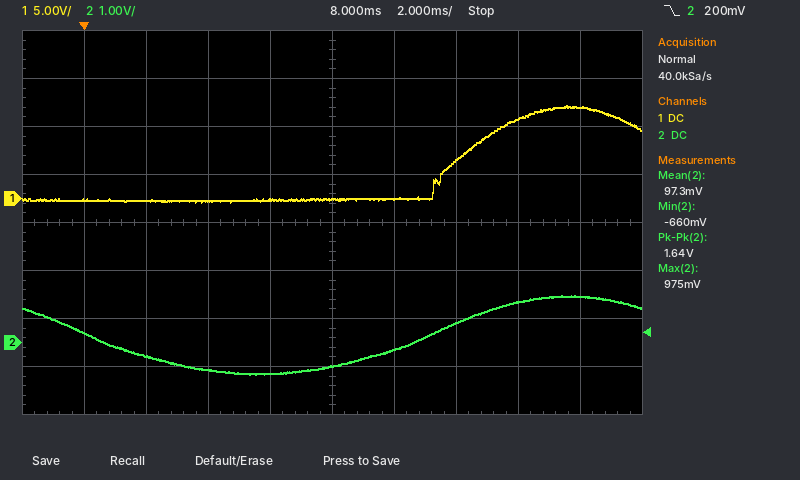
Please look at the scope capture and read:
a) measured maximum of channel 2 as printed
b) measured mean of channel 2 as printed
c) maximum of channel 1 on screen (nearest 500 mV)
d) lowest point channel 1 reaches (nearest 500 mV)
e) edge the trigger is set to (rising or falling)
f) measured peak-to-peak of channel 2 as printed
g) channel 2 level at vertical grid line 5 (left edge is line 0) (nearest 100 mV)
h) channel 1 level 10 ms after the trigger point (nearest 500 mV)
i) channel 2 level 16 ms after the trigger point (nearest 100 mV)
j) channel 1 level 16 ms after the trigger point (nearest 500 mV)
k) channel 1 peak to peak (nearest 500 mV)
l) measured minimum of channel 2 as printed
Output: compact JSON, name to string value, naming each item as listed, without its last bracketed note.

{"measured maximum of channel 2 as printed": "975 mV", "measured mean of channel 2 as printed": "97.3 mV", "maximum of channel 1 on screen": "9.5 V", "lowest point channel 1 reaches": "-500 mV", "edge the trigger is set to": "falling", "measured peak-to-peak of channel 2 as printed": "1.64 V", "channel 2 level at vertical grid line 5 (left edge is line 0)": "-500 mV", "channel 1 level 10 ms after the trigger point": "0.0 V", "channel 2 level 16 ms after the trigger point": "1.0 V", "channel 1 level 16 ms after the trigger point": "9.5 V", "channel 1 peak to peak": "10.0 V", "measured minimum of channel 2 as printed": "-660 mV"}
